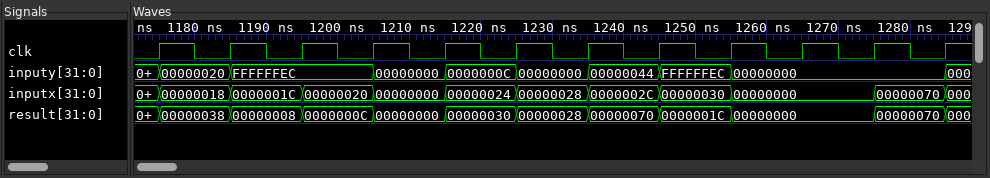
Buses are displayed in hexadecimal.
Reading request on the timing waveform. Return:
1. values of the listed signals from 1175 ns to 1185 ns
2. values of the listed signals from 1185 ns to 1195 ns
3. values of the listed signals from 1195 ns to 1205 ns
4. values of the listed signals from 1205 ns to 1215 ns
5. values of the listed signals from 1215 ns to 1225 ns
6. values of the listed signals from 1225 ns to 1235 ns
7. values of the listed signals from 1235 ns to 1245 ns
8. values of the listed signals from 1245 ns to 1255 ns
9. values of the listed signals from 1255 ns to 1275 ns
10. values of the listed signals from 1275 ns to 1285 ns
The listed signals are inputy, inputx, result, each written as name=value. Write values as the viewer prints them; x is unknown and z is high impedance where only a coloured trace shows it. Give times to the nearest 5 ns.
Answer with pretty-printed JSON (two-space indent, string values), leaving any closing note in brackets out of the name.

{
  "values of the listed signals from 1175 ns to 1185 ns": "inputy=00000020, inputx=00000018, result=00000038",
  "values of the listed signals from 1185 ns to 1195 ns": "inputy=FFFFFFEC, inputx=0000001C, result=00000008",
  "values of the listed signals from 1195 ns to 1205 ns": "inputy=FFFFFFEC, inputx=00000020, result=0000000C",
  "values of the listed signals from 1205 ns to 1215 ns": "inputy=00000000, inputx=00000000, result=00000000",
  "values of the listed signals from 1215 ns to 1225 ns": "inputy=0000000C, inputx=00000024, result=00000030",
  "values of the listed signals from 1225 ns to 1235 ns": "inputy=00000000, inputx=00000028, result=00000028",
  "values of the listed signals from 1235 ns to 1245 ns": "inputy=00000044, inputx=0000002C, result=00000070",
  "values of the listed signals from 1245 ns to 1255 ns": "inputy=FFFFFFEC, inputx=00000030, result=0000001C",
  "values of the listed signals from 1255 ns to 1275 ns": "inputy=00000000, inputx=00000000, result=00000000",
  "values of the listed signals from 1275 ns to 1285 ns": "inputy=00000000, inputx=00000070, result=00000070"
}
